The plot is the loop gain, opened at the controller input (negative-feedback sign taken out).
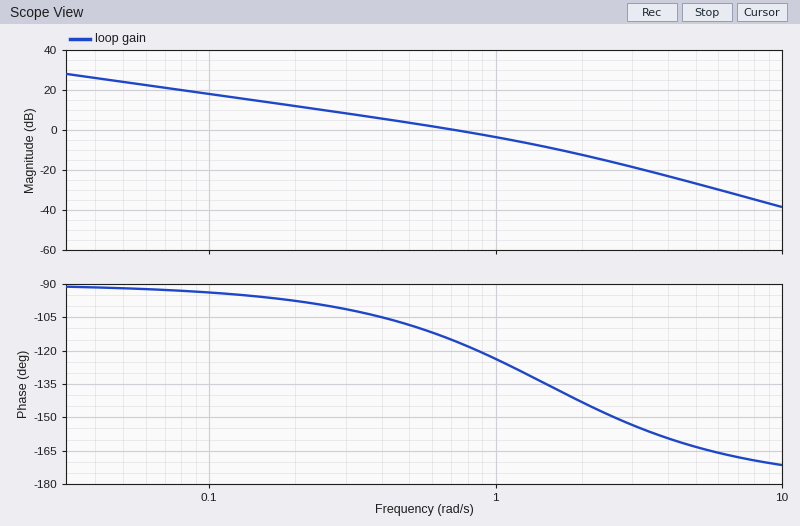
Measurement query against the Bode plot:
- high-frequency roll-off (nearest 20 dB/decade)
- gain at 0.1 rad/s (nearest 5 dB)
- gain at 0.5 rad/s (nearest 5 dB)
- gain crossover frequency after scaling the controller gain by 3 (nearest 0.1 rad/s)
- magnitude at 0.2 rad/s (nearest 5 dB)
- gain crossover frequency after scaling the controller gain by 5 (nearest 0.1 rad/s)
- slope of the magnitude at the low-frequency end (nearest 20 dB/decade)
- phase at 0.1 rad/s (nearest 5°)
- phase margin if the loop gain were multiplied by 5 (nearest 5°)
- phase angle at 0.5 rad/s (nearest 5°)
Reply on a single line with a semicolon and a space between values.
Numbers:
-40 dB/decade; 20 dB; 5 dB; 1.6 rad/s; 10 dB; 2.2 rad/s; -20 dB/decade; -95°; 35°; -110°
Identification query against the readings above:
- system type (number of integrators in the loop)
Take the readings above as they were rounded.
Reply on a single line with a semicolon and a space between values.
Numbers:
1
